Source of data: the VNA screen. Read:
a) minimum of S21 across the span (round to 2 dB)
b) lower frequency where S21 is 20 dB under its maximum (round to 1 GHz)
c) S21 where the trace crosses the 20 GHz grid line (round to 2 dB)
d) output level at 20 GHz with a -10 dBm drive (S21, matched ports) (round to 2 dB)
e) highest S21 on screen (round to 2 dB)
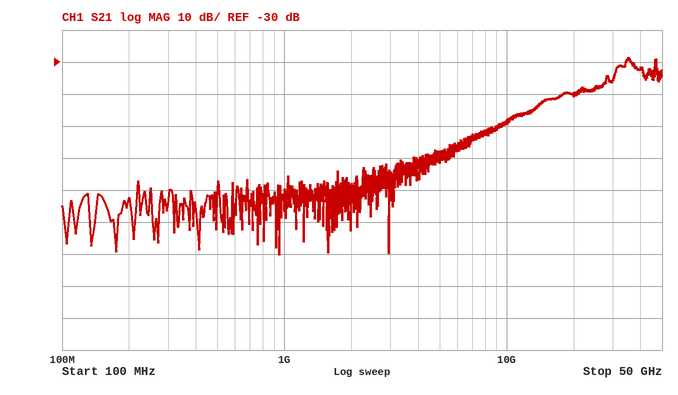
-90 dB
10 GHz
-40 dB
-50 dBm
-28 dB
